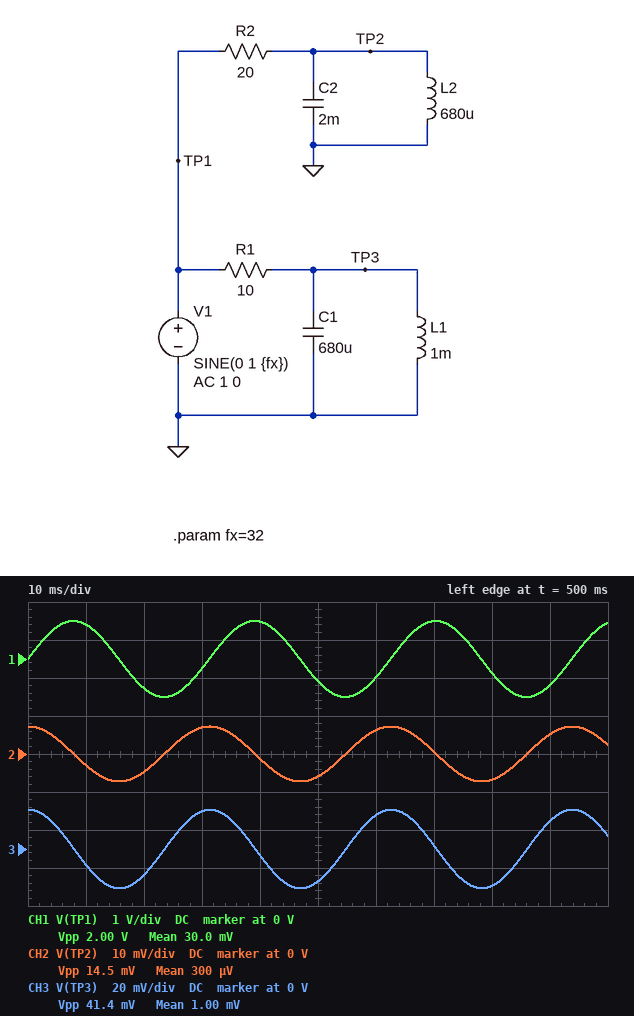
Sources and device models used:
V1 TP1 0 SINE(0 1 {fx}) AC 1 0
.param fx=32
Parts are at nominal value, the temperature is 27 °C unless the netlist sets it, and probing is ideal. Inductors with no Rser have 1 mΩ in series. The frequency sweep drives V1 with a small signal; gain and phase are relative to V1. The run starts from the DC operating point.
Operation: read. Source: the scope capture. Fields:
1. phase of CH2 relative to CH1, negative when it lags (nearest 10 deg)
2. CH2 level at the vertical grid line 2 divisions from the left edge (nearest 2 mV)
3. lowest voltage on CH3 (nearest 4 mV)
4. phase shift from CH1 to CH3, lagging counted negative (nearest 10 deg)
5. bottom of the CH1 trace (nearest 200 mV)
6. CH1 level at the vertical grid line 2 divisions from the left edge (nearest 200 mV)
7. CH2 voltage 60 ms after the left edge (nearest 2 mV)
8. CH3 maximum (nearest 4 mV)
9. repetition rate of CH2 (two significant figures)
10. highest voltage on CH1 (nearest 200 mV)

90 deg
-4 mV
-20 mV
90 deg
-1.0 V
-800 mV
6 mV
20 mV
32 Hz
1.0 V
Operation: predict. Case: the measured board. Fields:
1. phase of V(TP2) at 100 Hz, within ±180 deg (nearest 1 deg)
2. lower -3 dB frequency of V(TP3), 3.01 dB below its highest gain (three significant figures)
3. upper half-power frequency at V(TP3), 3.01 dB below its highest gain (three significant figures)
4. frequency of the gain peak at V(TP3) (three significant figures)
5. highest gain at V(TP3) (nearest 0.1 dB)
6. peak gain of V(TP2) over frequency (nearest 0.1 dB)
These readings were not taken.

87 deg
182 Hz
205 Hz
193 Hz
-0.1 dB
-0.5 dB
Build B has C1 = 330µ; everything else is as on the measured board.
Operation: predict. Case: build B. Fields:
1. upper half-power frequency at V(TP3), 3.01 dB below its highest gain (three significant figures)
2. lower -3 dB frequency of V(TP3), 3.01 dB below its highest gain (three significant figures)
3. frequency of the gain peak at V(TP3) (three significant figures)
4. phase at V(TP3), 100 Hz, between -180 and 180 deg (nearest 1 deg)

302 Hz
254 Hz
277 Hz
86 deg
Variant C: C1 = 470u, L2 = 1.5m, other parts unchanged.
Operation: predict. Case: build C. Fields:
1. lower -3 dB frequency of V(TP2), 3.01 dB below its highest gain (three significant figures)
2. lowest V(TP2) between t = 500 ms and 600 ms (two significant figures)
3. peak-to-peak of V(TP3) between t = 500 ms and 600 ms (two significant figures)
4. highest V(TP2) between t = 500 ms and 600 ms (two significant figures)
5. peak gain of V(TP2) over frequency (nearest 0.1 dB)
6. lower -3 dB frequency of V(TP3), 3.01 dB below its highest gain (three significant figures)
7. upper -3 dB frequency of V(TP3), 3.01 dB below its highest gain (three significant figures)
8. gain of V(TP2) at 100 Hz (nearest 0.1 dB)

89.9 Hz
-17 mV
41 mV
17 mV
-0.2 dB
216 Hz
250 Hz
-12.1 dB
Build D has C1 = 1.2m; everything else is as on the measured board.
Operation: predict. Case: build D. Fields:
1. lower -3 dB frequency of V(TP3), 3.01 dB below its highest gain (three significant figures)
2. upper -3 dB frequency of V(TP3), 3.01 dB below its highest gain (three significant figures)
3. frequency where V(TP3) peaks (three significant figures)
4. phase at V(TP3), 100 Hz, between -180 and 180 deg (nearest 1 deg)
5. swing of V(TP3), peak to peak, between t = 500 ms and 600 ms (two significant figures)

139 Hz
152 Hz
145 Hz
83 deg
42 mV
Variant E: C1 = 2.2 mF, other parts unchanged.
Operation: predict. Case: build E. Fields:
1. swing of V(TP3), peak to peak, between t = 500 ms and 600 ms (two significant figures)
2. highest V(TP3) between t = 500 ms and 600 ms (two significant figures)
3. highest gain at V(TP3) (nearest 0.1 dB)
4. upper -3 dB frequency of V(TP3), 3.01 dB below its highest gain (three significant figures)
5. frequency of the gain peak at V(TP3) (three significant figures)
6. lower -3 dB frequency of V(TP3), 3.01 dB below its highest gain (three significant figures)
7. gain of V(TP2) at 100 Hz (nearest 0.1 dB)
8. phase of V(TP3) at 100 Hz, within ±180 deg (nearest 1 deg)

44 mV
22 mV
-0.2 dB
111 Hz
107 Hz
104 Hz
-26.7 dB
64 deg
